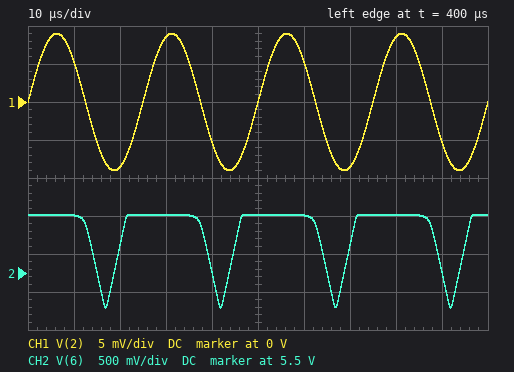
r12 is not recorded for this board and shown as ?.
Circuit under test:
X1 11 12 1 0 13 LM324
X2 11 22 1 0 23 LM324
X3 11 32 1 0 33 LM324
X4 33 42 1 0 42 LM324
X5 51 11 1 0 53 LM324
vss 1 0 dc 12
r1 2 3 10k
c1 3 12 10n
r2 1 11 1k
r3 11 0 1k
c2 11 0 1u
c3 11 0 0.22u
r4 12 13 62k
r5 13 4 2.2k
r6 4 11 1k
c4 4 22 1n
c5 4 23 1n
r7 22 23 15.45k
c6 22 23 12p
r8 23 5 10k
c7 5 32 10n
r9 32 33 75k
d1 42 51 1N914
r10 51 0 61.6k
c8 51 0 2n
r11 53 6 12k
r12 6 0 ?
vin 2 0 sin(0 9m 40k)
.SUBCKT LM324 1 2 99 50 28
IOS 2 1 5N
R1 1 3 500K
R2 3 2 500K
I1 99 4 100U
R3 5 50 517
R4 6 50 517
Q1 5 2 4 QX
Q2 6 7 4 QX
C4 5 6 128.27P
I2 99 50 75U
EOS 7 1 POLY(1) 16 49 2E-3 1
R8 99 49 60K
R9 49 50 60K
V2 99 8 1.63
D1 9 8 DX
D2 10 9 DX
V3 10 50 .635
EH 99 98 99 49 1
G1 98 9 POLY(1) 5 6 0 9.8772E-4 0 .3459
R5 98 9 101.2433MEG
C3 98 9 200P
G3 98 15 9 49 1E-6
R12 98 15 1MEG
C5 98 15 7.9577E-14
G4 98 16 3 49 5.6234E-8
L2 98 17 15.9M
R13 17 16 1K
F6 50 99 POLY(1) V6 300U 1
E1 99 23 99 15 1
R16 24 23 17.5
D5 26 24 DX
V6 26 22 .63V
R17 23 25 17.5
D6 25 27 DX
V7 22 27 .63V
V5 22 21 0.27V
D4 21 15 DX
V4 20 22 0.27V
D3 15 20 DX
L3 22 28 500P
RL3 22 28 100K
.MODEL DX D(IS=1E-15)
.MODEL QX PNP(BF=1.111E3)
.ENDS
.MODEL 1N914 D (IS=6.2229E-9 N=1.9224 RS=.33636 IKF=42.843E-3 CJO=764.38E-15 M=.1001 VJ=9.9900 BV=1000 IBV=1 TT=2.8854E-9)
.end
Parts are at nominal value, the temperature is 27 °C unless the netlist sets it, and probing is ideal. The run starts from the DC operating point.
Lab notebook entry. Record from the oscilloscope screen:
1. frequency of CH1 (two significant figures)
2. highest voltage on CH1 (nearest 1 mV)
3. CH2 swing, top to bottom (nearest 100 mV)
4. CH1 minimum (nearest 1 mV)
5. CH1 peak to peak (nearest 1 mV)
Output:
40 kHz
9 mV
1.2 V
-9 mV
18 mV
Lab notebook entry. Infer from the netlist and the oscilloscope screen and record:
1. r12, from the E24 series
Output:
16 kΩ
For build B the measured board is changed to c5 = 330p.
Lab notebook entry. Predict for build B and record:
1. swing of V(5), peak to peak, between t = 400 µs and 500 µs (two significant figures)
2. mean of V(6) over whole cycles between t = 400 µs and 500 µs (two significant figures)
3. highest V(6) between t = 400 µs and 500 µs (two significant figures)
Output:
60 mV
1.0 V
2.4 V
